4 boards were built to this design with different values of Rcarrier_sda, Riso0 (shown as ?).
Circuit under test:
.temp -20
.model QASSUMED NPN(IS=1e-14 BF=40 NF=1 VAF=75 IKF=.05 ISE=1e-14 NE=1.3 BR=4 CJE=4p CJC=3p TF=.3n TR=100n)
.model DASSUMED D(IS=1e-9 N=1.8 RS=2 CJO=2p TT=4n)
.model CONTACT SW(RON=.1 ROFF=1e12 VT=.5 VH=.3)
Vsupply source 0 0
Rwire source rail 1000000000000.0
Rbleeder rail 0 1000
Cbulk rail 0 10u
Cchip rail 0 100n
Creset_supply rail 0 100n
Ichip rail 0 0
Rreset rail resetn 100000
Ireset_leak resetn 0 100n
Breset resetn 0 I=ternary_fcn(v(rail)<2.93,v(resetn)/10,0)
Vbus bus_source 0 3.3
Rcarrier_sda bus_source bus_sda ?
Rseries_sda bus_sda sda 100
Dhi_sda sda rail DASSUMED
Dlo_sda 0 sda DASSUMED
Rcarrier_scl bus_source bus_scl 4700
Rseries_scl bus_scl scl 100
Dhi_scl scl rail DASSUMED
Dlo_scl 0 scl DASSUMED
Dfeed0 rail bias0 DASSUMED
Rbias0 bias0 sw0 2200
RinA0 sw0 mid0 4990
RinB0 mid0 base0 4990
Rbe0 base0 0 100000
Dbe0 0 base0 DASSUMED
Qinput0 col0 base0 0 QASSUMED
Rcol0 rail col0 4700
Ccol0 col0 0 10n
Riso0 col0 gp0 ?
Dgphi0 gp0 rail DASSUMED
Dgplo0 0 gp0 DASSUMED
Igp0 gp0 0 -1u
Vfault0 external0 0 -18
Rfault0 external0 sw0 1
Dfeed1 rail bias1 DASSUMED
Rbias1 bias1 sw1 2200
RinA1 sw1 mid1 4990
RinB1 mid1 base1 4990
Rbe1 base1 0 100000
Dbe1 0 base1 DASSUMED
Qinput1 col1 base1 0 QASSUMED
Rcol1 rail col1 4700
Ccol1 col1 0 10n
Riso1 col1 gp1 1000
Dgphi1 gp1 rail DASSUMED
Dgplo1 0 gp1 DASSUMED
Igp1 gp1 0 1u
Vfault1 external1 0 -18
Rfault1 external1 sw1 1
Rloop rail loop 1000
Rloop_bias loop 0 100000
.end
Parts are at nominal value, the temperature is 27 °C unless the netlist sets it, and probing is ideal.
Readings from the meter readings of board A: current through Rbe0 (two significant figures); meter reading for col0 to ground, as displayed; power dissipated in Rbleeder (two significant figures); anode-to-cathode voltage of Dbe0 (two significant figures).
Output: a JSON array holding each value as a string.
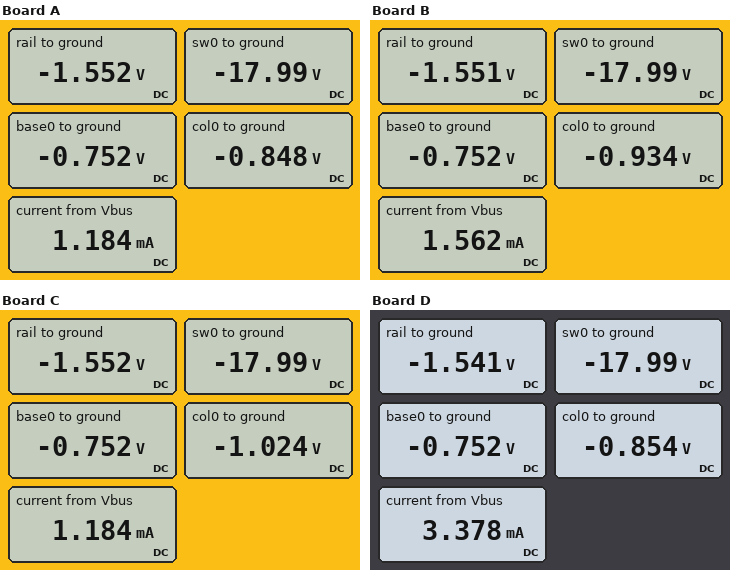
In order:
["7.5 µA", "-0.848 V", "2.4 mW", "750 mV"]
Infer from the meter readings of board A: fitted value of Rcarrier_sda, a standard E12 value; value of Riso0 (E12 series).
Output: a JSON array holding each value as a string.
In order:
["12 kΩ", "470 Ω"]
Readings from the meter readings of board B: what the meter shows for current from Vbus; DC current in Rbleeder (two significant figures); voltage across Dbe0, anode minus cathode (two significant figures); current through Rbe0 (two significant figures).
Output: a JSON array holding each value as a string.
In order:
["1.562 mA", "1.6 mA", "750 mV", "7.5 µA"]
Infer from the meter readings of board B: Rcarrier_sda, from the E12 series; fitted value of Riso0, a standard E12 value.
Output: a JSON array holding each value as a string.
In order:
["5.6 kΩ", "1.2 kΩ"]
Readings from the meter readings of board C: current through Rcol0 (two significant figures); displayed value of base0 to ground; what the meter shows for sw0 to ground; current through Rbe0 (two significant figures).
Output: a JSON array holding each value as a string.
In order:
["110 µA", "-0.752 V", "-17.99 V", "7.5 µA"]
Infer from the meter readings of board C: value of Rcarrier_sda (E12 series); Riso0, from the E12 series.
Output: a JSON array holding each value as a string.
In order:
["12 kΩ", "2.2 kΩ"]
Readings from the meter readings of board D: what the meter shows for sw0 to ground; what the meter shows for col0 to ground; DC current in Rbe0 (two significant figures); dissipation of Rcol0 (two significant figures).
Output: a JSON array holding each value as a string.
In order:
["-17.99 V", "-0.854 V", "7.5 µA", "100 µW"]
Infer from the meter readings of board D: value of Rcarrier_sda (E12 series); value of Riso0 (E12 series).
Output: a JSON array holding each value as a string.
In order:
["1.5 kΩ", "560 Ω"]
